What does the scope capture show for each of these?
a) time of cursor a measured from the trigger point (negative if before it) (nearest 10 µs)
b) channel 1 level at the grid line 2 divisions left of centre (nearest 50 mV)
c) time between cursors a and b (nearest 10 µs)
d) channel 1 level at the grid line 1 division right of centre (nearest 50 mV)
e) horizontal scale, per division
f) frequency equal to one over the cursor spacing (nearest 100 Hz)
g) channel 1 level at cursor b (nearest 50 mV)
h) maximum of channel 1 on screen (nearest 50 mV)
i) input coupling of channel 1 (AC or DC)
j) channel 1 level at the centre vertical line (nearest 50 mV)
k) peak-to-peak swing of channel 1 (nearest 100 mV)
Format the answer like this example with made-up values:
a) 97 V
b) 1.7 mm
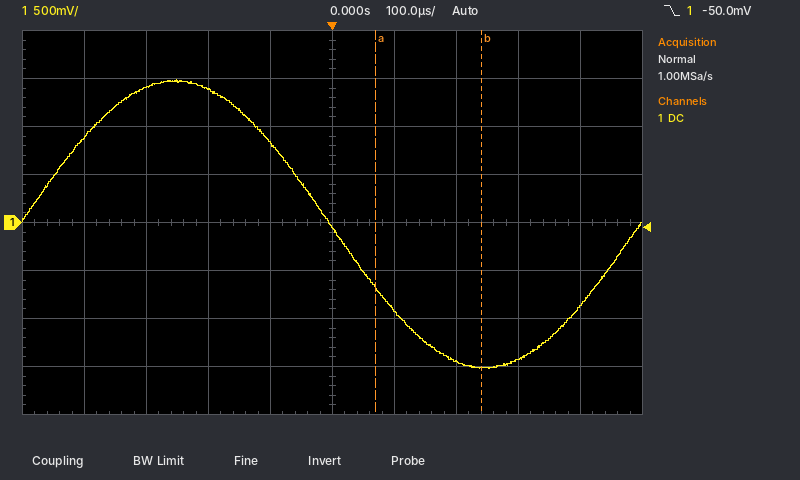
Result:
a) +70 µs
b) 1.40 V
c) 170 µs
d) -900 mV
e) 100 µs
f) 5.9 kHz
g) -1.50 V
h) 1.50 V
i) DC
j) -50 mV
k) 3.00 V
